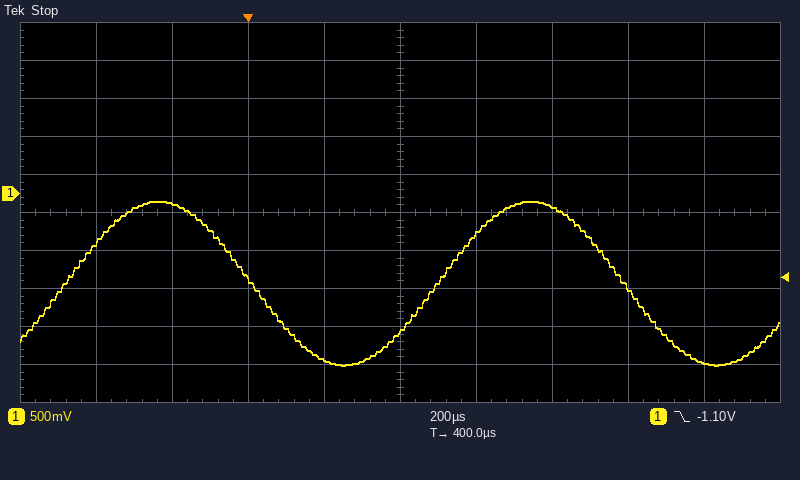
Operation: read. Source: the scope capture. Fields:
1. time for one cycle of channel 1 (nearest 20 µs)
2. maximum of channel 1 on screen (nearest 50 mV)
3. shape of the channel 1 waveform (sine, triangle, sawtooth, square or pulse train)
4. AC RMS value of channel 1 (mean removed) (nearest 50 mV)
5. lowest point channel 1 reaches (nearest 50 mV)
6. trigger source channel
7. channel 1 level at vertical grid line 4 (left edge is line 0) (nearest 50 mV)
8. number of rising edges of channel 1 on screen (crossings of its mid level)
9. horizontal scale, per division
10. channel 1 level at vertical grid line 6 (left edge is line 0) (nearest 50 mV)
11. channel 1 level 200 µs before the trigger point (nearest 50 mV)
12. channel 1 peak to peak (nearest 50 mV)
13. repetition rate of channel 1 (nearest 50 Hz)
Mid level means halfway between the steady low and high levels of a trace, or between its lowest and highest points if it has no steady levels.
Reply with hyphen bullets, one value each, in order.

- 980 µs
- -100 mV
- sine
- 750 mV
- -2.25 V
- channel 1
- -2.20 V
- 2
- 200 µs
- -550 mV
- -150 mV
- 2.15 V
- 1.00 kHz
